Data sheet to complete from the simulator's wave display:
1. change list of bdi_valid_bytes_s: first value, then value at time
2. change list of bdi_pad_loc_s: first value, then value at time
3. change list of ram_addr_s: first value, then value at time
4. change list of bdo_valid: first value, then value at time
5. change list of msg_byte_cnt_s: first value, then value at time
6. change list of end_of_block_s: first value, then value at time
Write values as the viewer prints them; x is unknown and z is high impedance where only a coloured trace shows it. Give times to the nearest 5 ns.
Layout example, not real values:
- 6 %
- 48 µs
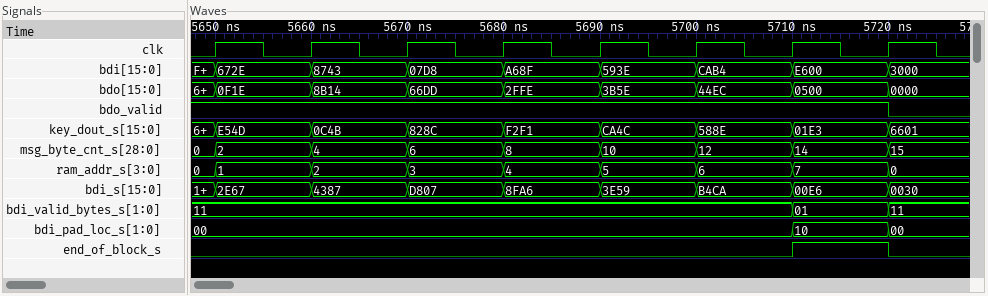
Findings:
- 11, 01 at 5710 ns, 11 at 5720 ns
- 00, 10 at 5710 ns, 00 at 5720 ns
- 0, 1 at 5650 ns, 2 at 5660 ns, 3 at 5670 ns, 4 at 5680 ns, 5 at 5690 ns, 6 at 5700 ns, 7 at 5710 ns, 0 at 5720 ns
- 1, 0 at 5720 ns
- 0, 2 at 5650 ns, 4 at 5660 ns, 6 at 5670 ns, 8 at 5680 ns, 10 at 5690 ns, 12 at 5700 ns, 14 at 5710 ns, 15 at 5720 ns
- 0, 1 at 5710 ns, 0 at 5720 ns
